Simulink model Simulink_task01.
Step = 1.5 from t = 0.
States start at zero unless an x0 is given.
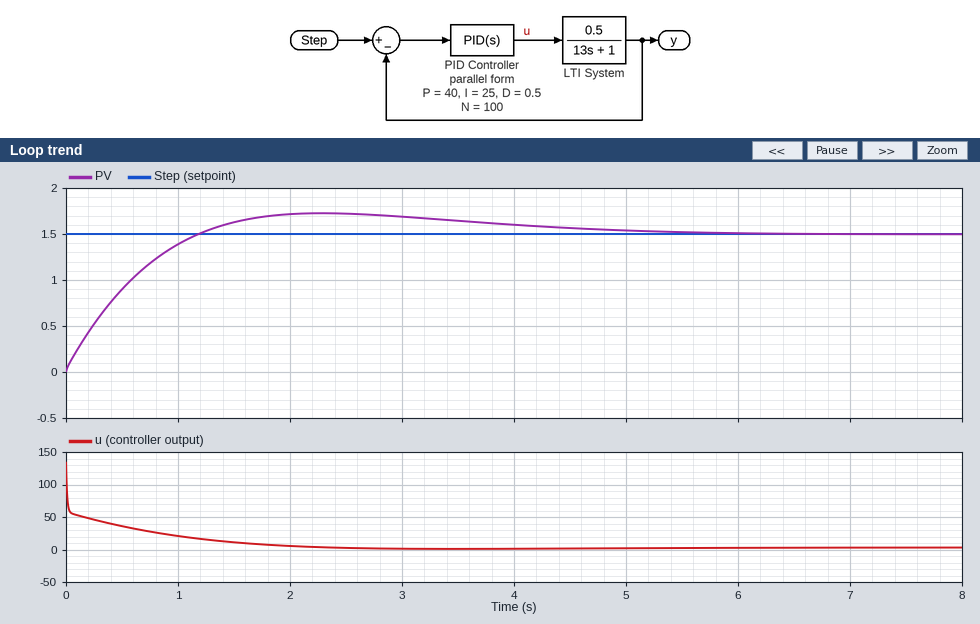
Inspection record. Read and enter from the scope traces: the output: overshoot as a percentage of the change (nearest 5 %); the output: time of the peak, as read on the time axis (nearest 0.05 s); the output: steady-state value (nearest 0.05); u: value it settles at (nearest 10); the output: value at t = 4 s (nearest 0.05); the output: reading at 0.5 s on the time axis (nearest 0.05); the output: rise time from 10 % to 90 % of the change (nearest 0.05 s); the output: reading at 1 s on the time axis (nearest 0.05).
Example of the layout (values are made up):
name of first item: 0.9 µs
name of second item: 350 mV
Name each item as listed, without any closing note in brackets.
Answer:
the output: overshoot as a percentage of the change: 15 %
the output: time of the peak, as read on the time axis: 2.30 s
the output: steady-state value: 1.50
u: value it settles at: 0
the output: value at t = 4 s: 1.60
the output: reading at 0.5 s on the time axis: 0.90
the output: rise time from 10 % to 90 % of the change: 0.90 s
the output: reading at 1 s on the time axis: 1.40
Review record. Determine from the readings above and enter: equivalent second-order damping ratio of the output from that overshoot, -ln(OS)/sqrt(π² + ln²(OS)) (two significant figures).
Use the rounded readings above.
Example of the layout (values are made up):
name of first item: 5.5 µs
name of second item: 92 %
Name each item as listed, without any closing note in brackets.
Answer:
equivalent second-order damping ratio of the output from that overshoot, -ln(OS)/sqrt(π² + ln²(OS)): 0.52
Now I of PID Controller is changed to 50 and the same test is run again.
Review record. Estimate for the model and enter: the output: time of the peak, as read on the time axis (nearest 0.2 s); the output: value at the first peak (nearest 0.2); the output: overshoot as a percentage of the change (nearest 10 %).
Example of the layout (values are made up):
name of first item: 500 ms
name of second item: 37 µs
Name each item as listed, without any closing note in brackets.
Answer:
the output: time of the peak, as read on the time axis: 1.8 s
the output: value at the first peak: 1.8
the output: overshoot as a percentage of the change: 20 %
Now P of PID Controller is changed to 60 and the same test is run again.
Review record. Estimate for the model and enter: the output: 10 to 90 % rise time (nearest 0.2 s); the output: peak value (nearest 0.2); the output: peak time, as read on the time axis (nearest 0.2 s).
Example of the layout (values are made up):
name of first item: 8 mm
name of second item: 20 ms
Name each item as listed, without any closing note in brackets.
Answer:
the output: 10 to 90 % rise time: 0.8 s
the output: peak value: 1.6
the output: peak time, as read on the time axis: 2.0 s
